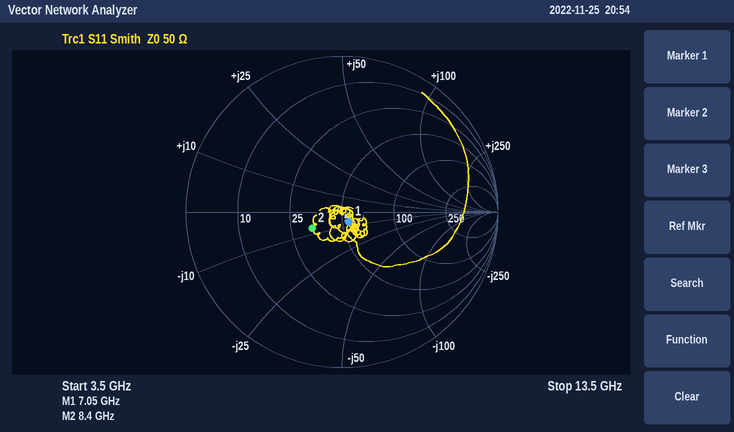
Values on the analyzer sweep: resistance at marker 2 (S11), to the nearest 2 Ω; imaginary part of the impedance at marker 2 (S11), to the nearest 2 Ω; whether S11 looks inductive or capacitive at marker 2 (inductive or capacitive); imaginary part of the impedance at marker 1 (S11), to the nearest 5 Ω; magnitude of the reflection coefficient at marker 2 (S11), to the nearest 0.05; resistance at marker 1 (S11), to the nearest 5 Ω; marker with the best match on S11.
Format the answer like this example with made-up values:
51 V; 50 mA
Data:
34 Ω; -8 Ω; capacitive; -5 Ω; 0.20; 55 Ω; marker 1
